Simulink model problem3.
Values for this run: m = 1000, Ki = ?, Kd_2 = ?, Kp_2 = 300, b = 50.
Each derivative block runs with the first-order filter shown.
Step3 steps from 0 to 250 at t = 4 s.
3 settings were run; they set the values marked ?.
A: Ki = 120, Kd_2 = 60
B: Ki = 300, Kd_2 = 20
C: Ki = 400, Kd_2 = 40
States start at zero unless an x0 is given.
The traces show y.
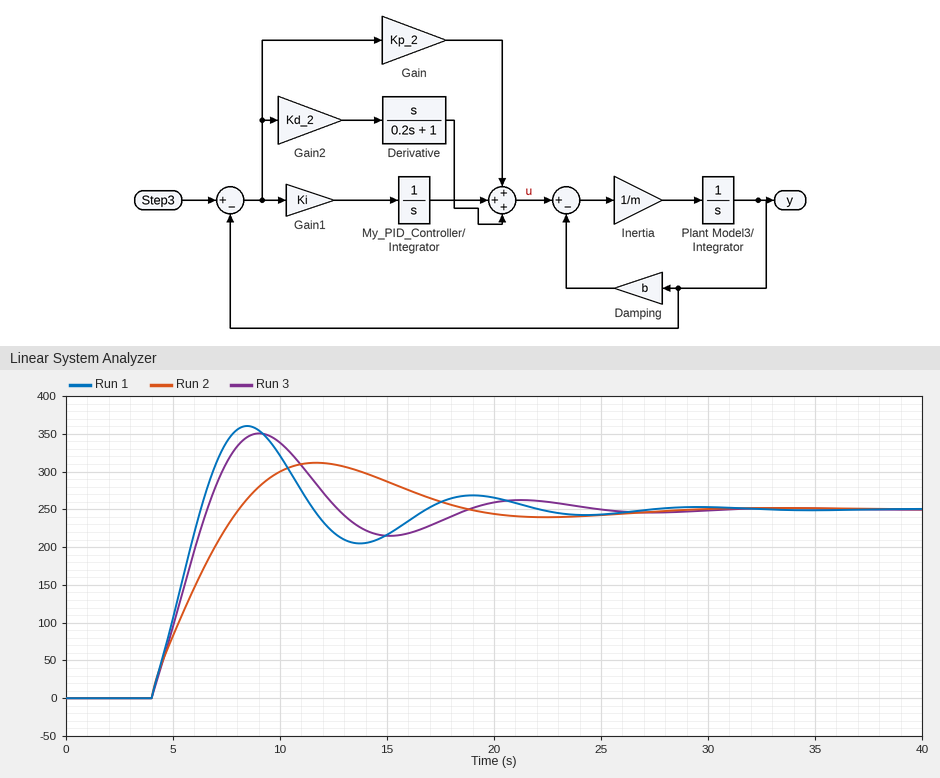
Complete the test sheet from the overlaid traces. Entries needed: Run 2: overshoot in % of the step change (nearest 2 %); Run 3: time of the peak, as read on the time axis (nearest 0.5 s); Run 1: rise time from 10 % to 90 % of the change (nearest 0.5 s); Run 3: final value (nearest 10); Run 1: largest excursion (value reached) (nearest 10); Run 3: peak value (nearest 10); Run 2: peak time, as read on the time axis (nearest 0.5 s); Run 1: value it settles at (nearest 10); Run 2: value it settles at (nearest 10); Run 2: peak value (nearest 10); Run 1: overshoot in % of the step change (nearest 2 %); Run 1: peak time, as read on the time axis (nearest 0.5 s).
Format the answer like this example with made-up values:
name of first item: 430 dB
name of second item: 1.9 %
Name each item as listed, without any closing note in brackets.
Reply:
Run 2: overshoot in % of the step change: 24 %
Run 3: time of the peak, as read on the time axis: 9.0 s
Run 1: rise time from 10 % to 90 % of the change: 2.0 s
Run 3: final value: 250
Run 1: largest excursion (value reached): 360
Run 3: peak value: 350
Run 2: peak time, as read on the time axis: 11.5 s
Run 1: value it settles at: 250
Run 2: value it settles at: 250
Run 2: peak value: 310
Run 1: overshoot in % of the step change: 44 %
Run 1: peak time, as read on the time axis: 8.5 s
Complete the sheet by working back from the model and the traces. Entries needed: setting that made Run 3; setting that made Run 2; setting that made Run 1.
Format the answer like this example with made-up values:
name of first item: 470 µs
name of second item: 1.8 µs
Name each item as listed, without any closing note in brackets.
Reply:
setting that made Run 3: B
setting that made Run 2: A
setting that made Run 1: C
